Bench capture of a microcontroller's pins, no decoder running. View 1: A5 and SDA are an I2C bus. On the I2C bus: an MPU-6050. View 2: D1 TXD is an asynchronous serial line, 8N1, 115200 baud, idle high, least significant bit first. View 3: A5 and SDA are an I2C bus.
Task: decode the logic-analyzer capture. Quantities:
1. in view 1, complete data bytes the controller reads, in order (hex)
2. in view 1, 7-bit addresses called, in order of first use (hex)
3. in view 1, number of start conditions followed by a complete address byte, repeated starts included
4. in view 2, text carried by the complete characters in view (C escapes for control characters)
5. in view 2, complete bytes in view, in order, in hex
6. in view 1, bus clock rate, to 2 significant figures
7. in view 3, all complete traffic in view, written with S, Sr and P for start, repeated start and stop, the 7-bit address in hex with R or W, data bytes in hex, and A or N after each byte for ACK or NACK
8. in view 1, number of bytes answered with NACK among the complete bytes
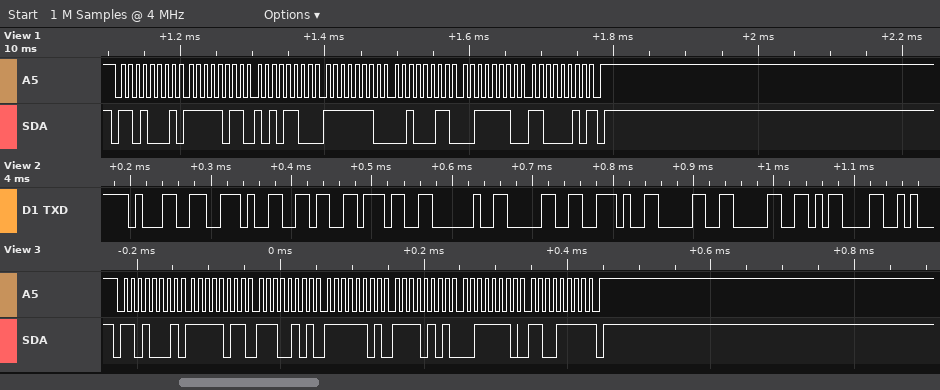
FB AC FE 23 3E C2
0x68
1
"1.67 0.00\r"
0x31 0x2E 0x36 0x37 0x20 0x30 0x2E 0x30 0x30 0x0D
100 kHz
S 68R A FB A E5 A FD A F5 A 3E A CF N P
1
